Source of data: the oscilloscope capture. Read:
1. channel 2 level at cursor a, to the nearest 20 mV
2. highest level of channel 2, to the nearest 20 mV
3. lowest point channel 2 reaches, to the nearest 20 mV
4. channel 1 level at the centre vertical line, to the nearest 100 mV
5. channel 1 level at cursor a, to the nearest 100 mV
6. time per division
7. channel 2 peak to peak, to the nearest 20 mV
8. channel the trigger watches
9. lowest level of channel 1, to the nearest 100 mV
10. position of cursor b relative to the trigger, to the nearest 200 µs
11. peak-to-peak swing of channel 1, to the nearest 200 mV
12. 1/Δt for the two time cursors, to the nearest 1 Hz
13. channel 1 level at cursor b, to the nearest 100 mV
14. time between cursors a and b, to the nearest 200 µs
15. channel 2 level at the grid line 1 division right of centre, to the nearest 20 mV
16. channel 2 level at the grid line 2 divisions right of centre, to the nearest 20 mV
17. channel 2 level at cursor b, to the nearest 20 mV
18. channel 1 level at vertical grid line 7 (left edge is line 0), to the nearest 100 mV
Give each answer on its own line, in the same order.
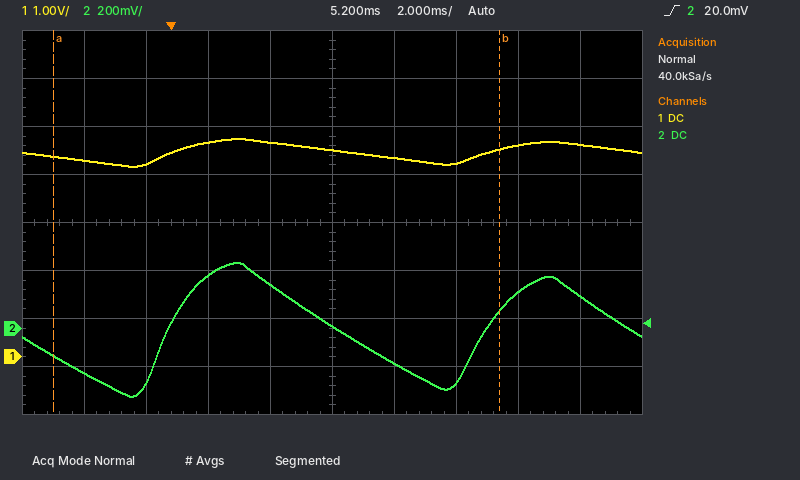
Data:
-120 mV
280 mV
-280 mV
4.3 V
4.2 V
2 ms
560 mV
channel 2
4.0 V
+10.6 ms
600 mV
69 Hz
4.3 V
14.4 ms
-140 mV
-220 mV
80 mV
4.0 V
